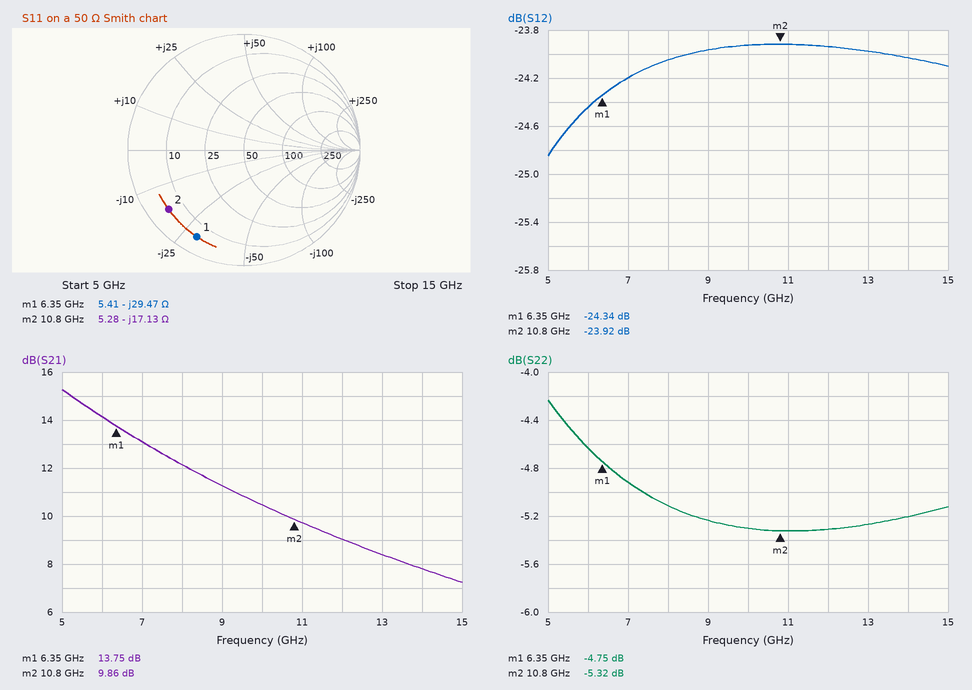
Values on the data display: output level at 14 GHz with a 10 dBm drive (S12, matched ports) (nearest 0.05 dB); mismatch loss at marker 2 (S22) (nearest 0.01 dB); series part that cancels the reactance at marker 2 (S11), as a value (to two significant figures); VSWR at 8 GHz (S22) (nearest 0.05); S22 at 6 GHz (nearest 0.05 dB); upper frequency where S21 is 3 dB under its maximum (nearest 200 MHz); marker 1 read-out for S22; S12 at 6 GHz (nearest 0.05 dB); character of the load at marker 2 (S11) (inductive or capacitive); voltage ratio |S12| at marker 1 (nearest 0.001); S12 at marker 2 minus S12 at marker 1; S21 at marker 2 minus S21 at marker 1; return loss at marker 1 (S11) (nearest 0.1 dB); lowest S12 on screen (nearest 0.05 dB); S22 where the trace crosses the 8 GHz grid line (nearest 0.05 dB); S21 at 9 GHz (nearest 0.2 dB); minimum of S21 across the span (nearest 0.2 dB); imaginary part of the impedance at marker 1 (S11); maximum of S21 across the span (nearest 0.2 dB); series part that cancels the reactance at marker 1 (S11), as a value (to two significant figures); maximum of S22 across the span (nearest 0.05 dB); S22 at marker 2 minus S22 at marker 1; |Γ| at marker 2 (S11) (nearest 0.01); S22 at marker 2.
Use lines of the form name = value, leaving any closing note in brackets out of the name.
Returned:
output level at 14 GHz with a 10 dBm drive (S12, matched ports) = -14.05 dBm
mismatch loss at marker 2 (S22) = 1.51 dB
series part that cancels the reactance at marker 2 (S11), as a value = 250 pH
VSWR at 8 GHz (S22) = 3.50
S22 at 6 GHz = -4.65 dB
upper frequency where S21 is 3 dB under its maximum = 7.8 GHz
marker 1 read-out for S22 = -4.75 dB
S12 at 6 GHz = -24.45 dB
character of the load at marker 2 (S11) = capacitive
voltage ratio |S12| at marker 1 = 0.061
S12 at marker 2 minus S12 at marker 1 = 0.42 dB
S21 at marker 2 minus S21 at marker 1 = -3.89 dB
return loss at marker 1 (S11) = 1.4 dB
lowest S12 on screen = -24.85 dB
S22 where the trace crosses the 8 GHz grid line = -5.10 dB
S21 at 9 GHz = 11.2 dB
minimum of S21 across the span = 7.2 dB
imaginary part of the impedance at marker 1 = -29.47 Ω
maximum of S21 across the span = 15.2 dB
series part that cancels the reactance at marker 1 (S11), as a value = 740 pH
maximum of S22 across the span = -4.25 dB
S22 at marker 2 minus S22 at marker 1 = -0.57 dB
|Γ| at marker 2 (S11) = 0.83
S22 at marker 2 = -5.32 dB
